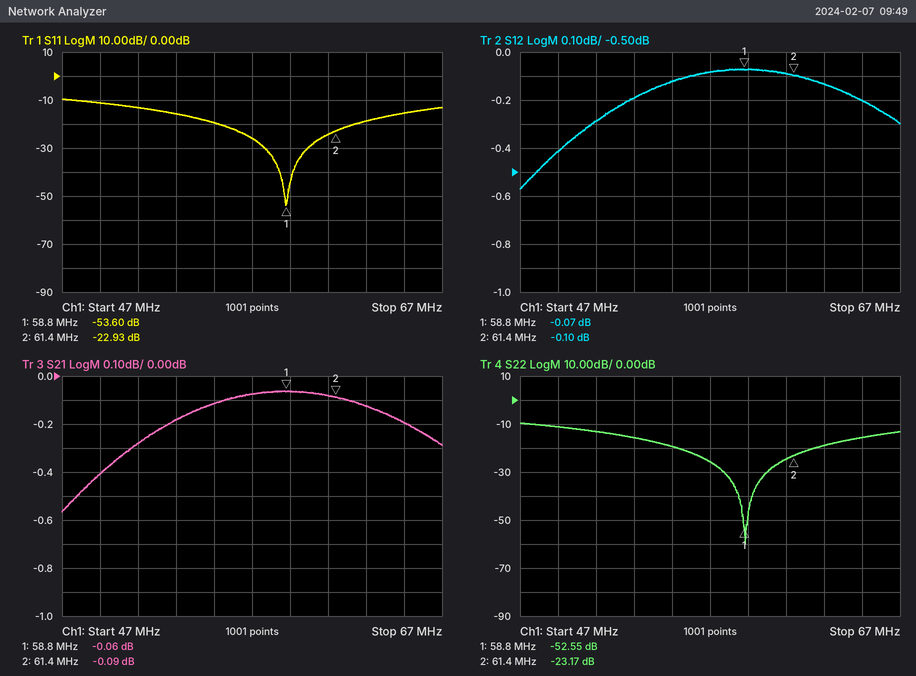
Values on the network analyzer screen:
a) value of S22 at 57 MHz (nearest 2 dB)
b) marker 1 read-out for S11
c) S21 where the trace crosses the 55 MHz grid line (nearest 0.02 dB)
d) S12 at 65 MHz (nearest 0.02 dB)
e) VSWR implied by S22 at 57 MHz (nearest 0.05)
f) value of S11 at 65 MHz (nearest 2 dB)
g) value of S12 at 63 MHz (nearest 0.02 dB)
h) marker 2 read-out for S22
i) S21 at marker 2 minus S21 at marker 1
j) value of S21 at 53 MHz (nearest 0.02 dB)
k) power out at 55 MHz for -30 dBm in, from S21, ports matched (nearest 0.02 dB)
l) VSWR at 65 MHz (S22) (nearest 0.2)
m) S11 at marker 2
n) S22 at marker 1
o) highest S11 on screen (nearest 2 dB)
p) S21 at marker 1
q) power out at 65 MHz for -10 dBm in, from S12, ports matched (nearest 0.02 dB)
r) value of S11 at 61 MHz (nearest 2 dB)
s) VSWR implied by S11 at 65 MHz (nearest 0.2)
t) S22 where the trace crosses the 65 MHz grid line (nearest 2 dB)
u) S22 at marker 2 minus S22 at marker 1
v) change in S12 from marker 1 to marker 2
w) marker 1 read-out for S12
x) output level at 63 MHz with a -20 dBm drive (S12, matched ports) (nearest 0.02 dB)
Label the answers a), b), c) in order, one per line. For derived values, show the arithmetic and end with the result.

a) -26 dB
b) -53.60 dB
c) -0.12 dB
d) -0.20 dB
e) |Γ| = 10^(-26/20) = 0.0501; VSWR = (1 + 0.0501)/(1 − 0.0501) ≈ 1.11, so 1.10 to the nearest 0.05
f) -16 dB
g) -0.14 dB
h) -23.17 dB
i) -0.09 − (-0.06) = -0.03 dB
j) -0.18 dB
k) -30 dBm + (-0.12 dB) = -30.12 dBm
l) |Γ| = 10^(-16/20) = 0.1585; VSWR = (1 + 0.1585)/(1 − 0.1585) ≈ 1.4
m) -22.93 dB
n) -52.55 dB
o) -10 dB
p) -0.06 dB
q) -10 dBm + (-0.20 dB) = -10.20 dBm
r) -24 dB
s) |Γ| = 10^(-16/20) = 0.1585; VSWR = (1 + 0.1585)/(1 − 0.1585) ≈ 1.4
t) -16 dB
u) -23.17 − (-52.55) = 29.38 dB
v) -0.1 − (-0.07) = -0.03 dB
w) -0.07 dB
x) -20 dBm + (-0.14 dB) = -20.14 dBm
